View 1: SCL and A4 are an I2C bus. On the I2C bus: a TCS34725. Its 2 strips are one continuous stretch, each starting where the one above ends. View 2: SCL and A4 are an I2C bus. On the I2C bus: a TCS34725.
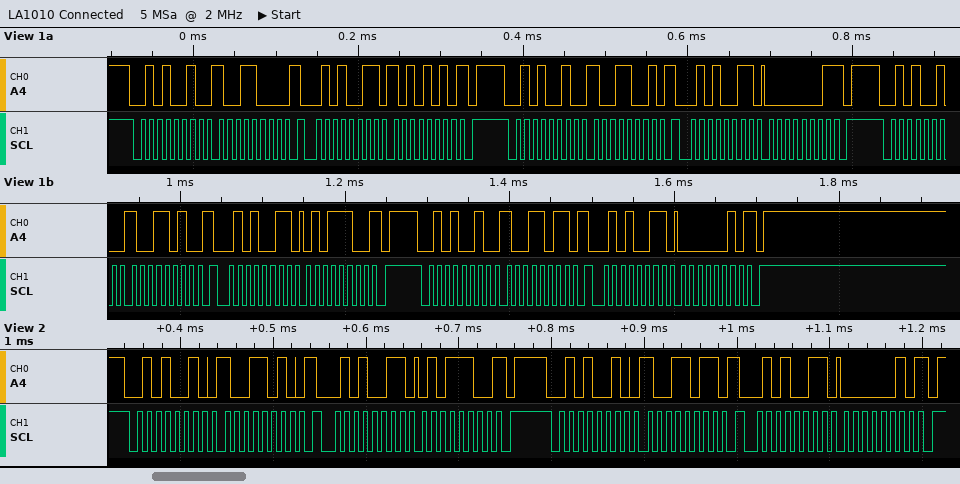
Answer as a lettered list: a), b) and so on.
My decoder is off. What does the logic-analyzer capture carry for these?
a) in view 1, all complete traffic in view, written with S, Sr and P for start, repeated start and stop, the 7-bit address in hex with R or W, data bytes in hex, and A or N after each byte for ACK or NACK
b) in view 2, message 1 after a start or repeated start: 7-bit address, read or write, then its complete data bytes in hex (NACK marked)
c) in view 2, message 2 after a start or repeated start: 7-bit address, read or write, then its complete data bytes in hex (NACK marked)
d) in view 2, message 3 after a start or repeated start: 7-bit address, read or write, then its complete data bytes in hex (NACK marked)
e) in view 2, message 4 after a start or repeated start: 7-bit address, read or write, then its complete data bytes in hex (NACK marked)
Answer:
a) S 29W A 98 A Sr 29R A AA N P S 29W A 99 A Sr 29R A 01 N P S 29W A 9A A Sr 29R A 5C N P S 29W A 9B A Sr 29R A 02 N P
b) 0x29 write: 9A
c) 0x29 read: 5C NACK
d) 0x29 write: 9B
e) 0x29 read: 02 NACK
